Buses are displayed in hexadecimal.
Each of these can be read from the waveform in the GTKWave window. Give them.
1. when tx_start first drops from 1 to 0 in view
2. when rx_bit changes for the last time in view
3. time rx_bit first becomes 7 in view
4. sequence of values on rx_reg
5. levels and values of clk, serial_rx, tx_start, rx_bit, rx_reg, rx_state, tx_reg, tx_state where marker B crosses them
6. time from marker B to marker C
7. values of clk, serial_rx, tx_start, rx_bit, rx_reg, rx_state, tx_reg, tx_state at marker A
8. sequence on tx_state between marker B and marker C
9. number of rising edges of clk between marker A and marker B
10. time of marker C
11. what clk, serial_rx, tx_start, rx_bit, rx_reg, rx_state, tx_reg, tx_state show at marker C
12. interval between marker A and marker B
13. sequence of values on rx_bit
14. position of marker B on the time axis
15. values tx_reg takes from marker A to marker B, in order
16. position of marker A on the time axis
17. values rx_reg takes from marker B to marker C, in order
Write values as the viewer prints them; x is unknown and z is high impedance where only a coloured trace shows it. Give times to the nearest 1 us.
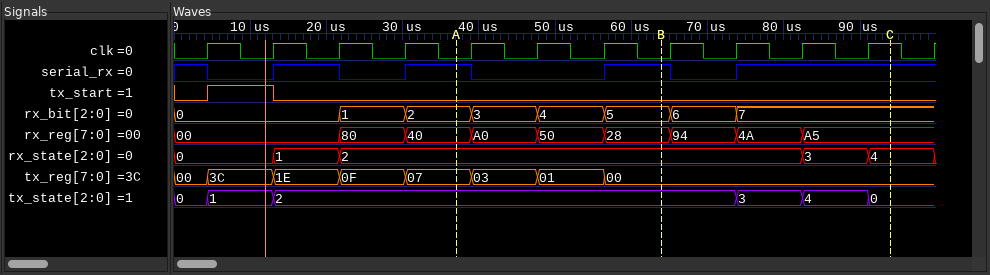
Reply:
13 us
74 us
74 us
00, 80, 40, A0, 50, 28, 94, 4A, A5
clk=0, serial_rx=1, tx_start=0, rx_bit=5, rx_reg=28, rx_state=2, tx_reg=00, tx_state=2
30 us
clk=0, serial_rx=1, tx_start=0, rx_bit=2, rx_reg=40, rx_state=2, tx_reg=07, tx_state=2
2, 3, 4, 0
3
94 us
clk=1, serial_rx=1, tx_start=0, rx_bit=7, rx_reg=A5, rx_state=4, tx_reg=00, tx_state=0
27 us
0, 1, 2, 3, 4, 5, 6, 7
64 us
07, 03, 01, 00
37 us
28, 94, 4A, A5
